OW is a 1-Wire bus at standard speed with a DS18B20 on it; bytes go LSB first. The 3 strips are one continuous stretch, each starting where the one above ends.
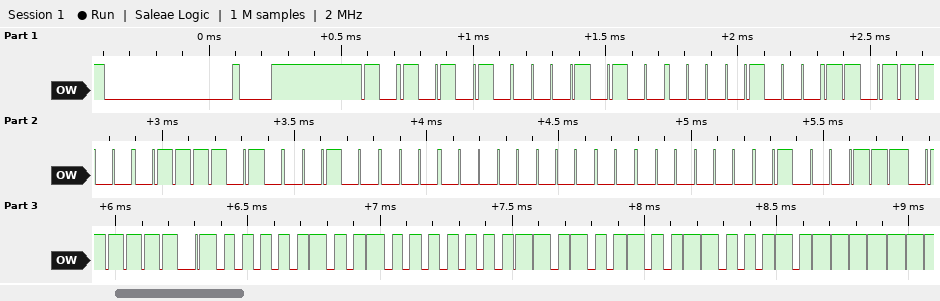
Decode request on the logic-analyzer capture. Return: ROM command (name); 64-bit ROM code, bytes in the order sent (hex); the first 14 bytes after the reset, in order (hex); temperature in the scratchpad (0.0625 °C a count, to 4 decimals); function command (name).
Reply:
Match ROM
28 10 3B 5E 04 00 00 E2
55 28 10 3B 5E 04 00 00 E2 BE 20 01 4B 46
18.0000 °C
Read Scratchpad
